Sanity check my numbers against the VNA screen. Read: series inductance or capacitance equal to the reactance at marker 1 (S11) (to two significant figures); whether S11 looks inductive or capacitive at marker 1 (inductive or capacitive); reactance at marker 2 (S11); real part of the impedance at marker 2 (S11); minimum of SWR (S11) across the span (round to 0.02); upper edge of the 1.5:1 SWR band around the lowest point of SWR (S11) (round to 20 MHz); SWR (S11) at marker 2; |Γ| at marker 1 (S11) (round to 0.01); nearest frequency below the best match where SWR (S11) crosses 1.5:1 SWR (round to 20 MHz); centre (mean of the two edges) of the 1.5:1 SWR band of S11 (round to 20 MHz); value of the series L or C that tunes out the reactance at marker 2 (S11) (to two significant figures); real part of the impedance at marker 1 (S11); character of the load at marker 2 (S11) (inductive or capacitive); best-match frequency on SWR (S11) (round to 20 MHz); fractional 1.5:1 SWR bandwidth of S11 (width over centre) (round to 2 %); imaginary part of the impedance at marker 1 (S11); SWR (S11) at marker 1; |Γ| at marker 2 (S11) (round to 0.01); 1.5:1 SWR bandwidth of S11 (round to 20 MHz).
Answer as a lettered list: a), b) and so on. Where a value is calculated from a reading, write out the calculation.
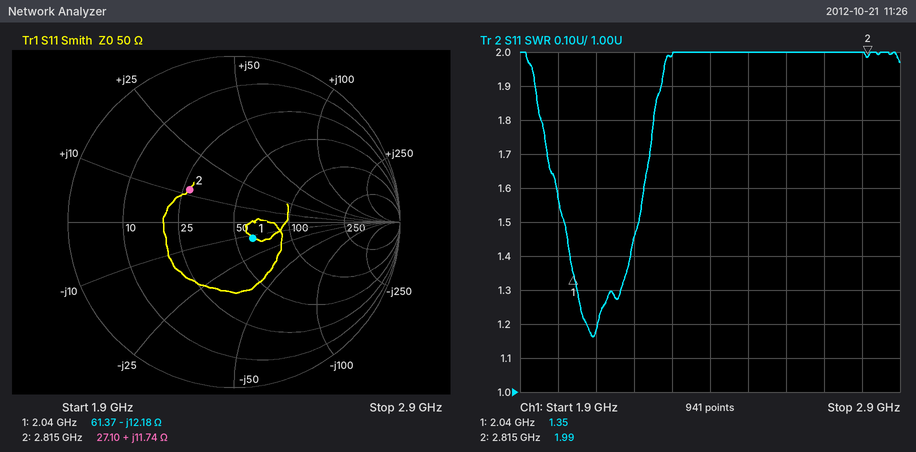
a) C = 1/(2π × 2.04 GHz × 12.18 Ω) ≈ 6.4 pF
b) capacitive
c) +11.74 Ω
d) 27.10 Ω
e) 1.16
f) 2.22 GHz
g) 1.99
h) 0.15
i) 2.02 GHz
j) 2.12 GHz
k) C = 1/(2π × 2.815 GHz × 11.74 Ω) ≈ 4.8 pF
l) 61.37 Ω
m) inductive
n) 2.10 GHz
o) 200 MHz / 2.12 GHz ≈ 9.43 %, so 10 % to the nearest 2 %
p) -12.18 Ω
q) 1.35
r) 0.33
s) 2.22 GHz − 2.02 GHz = 200 MHz
